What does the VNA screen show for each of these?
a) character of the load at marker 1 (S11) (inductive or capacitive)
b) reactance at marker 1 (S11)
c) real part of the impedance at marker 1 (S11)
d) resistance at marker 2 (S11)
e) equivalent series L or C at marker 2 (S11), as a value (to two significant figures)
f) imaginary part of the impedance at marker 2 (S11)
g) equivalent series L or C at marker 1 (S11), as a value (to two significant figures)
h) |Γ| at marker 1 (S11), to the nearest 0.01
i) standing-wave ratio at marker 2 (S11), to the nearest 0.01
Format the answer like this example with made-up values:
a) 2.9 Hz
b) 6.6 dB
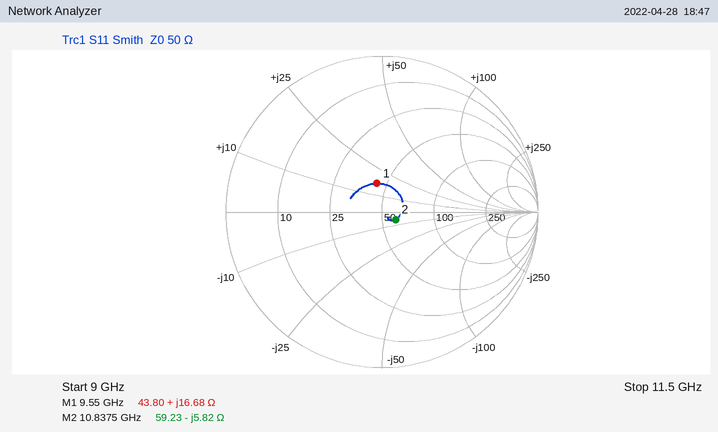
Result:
a) inductive
b) +16.68 Ω
c) 43.80 Ω
d) 59.23 Ω
e) 2.5 pF
f) -5.82 Ω
g) 280 pH
h) 0.19
i) 1.22
